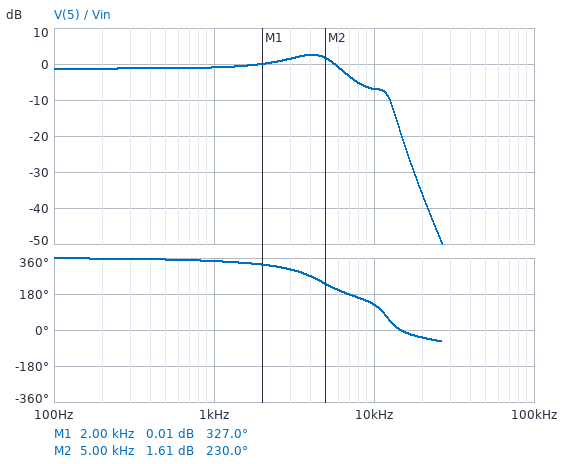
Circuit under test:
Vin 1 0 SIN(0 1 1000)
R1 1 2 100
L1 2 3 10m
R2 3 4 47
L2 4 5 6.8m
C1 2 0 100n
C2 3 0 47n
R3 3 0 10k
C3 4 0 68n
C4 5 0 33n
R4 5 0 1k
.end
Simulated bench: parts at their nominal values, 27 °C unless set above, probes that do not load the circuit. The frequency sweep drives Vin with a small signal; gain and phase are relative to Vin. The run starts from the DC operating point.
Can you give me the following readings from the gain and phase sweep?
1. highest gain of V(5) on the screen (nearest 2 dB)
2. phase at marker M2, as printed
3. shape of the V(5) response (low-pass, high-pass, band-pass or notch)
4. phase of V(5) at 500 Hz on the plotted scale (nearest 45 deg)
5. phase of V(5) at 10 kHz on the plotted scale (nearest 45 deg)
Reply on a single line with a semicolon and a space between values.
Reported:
2 dB; 230.0 deg; low-pass; 360 deg; 135 deg
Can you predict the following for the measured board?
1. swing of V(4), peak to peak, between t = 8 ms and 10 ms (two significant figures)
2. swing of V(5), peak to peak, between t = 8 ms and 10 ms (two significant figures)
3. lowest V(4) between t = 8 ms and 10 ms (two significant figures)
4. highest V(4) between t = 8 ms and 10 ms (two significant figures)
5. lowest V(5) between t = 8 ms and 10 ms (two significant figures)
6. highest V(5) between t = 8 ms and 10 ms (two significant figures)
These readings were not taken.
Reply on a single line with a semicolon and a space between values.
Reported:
1.8 V; 1.8 V; -890 mV; 890 mV; -900 mV; 900 mV
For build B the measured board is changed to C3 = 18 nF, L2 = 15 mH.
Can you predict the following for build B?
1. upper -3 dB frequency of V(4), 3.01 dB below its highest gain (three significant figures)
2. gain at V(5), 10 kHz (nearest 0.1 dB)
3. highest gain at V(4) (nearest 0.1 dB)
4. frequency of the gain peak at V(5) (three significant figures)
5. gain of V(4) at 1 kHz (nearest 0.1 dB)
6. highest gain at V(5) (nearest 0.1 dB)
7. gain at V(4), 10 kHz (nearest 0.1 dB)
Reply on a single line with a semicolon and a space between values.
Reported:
10.6 kHz; -1.0 dB; 2.4 dB; 4.73 kHz; -1.1 dB; 2.3 dB; 1.6 dB
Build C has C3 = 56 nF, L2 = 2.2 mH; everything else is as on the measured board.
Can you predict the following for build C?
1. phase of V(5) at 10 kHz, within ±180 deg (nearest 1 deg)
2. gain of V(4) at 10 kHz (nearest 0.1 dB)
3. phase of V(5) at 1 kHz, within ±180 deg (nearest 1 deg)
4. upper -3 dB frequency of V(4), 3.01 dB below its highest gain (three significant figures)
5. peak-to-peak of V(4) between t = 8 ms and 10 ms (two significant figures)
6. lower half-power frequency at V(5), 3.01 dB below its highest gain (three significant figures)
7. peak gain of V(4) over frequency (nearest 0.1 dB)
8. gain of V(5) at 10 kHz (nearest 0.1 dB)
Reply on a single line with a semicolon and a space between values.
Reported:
158 deg; -14.6 dB; -13 deg; 5.68 kHz; 1.8 V; 1.68 kHz; 2.1 dB; -11.8 dB
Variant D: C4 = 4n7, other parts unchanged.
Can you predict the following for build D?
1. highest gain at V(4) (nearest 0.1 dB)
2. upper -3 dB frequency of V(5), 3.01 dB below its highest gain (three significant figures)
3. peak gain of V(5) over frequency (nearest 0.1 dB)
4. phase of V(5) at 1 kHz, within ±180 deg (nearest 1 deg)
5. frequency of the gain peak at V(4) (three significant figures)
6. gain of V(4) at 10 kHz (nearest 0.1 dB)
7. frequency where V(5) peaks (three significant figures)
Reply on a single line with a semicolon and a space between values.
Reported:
2.6 dB; 6.26 kHz; 2.7 dB; -14 deg; 4.71 kHz; -11.8 dB; 4.72 kHz
